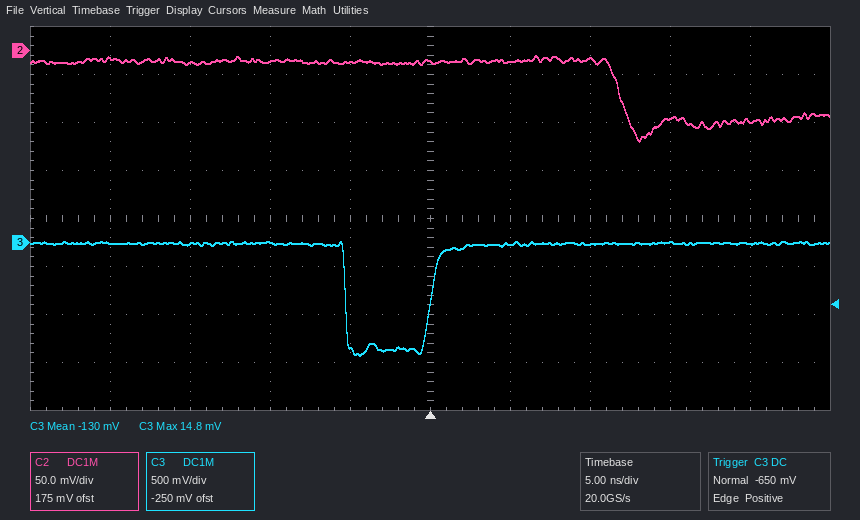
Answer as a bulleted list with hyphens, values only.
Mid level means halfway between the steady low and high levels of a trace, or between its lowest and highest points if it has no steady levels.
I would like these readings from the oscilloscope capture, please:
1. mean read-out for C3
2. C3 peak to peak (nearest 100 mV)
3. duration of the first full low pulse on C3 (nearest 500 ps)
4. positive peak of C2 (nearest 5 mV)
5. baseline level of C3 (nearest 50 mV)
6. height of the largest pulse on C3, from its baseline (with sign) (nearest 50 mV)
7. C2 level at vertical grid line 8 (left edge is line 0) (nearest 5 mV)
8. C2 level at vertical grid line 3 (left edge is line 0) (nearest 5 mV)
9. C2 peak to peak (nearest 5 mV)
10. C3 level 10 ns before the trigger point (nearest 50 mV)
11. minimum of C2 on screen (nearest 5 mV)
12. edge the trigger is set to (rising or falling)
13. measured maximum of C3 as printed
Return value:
- -130 mV
- 1.20 V
- 5.5 ns
- -5 mV
- 0 mV
- -1.15 V
- -70 mV
- -10 mV
- 90 mV
- 0 mV
- -95 mV
- rising
- 14.8 mV
